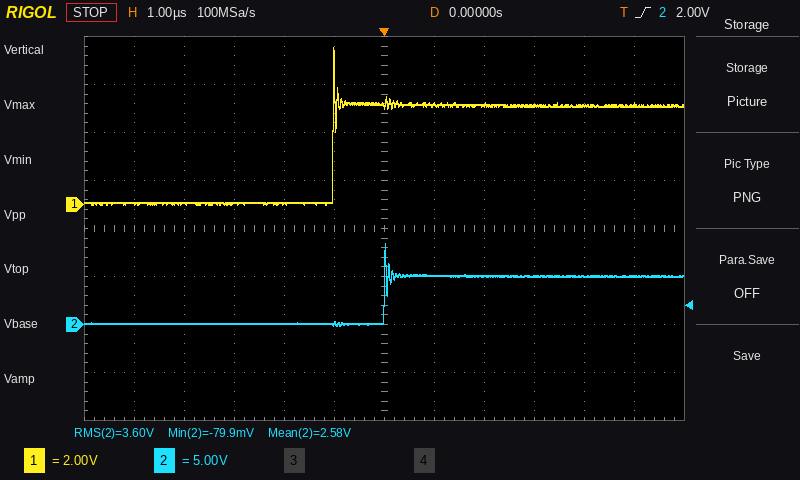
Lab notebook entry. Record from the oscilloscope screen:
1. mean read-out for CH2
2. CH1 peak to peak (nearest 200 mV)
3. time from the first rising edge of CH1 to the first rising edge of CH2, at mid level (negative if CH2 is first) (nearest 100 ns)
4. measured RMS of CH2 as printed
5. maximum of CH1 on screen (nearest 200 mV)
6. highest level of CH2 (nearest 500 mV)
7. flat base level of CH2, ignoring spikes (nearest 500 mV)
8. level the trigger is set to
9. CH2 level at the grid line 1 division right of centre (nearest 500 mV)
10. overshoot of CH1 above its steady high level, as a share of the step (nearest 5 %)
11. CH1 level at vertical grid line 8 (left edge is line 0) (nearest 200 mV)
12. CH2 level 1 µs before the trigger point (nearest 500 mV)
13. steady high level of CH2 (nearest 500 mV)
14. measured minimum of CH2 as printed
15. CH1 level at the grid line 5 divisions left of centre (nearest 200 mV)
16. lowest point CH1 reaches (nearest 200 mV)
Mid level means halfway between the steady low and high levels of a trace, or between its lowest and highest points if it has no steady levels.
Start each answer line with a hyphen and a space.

- 2.58 V
- 6.6 V
- +1.0 µs
- 3.60 V
- 6.6 V
- 8.5 V
- 0.0 V
- 2.00 V
- 5.0 V
- 60 %
- 4.2 V
- 0.0 V
- 5.0 V
- -79.9 mV
- 0.0 V
- 0.0 V
